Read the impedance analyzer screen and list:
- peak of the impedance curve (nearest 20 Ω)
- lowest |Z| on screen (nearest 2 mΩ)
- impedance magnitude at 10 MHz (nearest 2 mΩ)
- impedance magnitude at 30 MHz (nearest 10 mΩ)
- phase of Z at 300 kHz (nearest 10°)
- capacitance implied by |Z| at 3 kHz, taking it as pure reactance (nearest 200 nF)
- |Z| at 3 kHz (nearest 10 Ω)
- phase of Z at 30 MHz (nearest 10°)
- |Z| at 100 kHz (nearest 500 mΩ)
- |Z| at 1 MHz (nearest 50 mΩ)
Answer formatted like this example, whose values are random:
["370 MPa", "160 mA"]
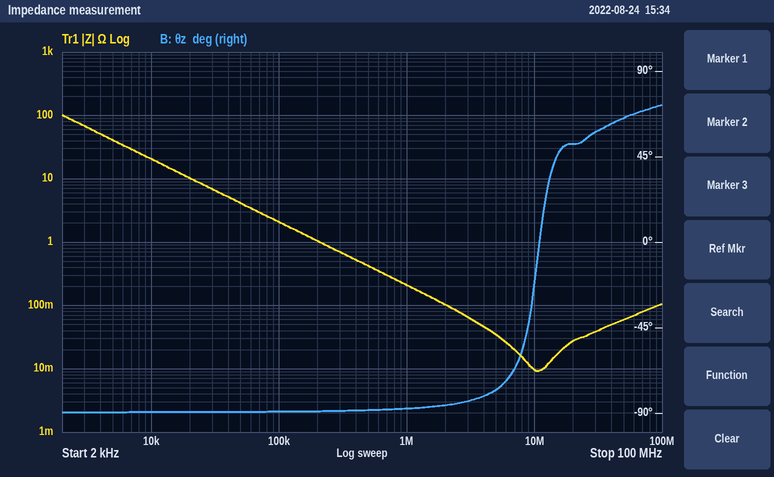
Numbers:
["100 Ω", "10 mΩ", "10 mΩ", "40 mΩ", "-90°", "800 nF", "70 Ω", "60°", "2.0 Ω", "200 mΩ"]
